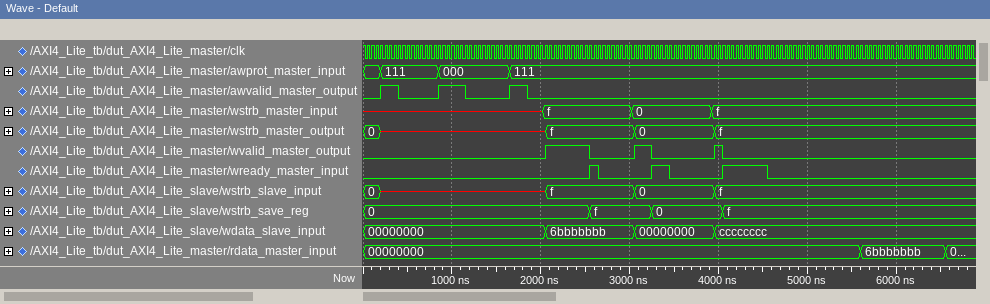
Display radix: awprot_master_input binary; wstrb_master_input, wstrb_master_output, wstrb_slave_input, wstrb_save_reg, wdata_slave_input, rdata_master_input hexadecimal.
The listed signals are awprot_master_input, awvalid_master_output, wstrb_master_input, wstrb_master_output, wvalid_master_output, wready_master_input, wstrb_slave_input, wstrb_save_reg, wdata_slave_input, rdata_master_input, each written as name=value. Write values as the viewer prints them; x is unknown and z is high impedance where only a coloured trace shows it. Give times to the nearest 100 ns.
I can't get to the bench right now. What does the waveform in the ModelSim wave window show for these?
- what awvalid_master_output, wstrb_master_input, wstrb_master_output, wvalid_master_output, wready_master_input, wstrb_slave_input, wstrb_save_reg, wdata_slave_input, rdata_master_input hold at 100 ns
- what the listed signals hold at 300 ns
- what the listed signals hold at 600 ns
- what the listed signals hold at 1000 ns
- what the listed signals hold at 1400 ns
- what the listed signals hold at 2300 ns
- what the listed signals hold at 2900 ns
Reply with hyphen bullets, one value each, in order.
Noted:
- awvalid_master_output=0, wstrb_master_input=x, wstrb_master_output=0, wvalid_master_output=0, wready_master_input=0, wstrb_slave_input=0, wstrb_save_reg=0, wdata_slave_input=00000000, rdata_master_input=00000000
- awprot_master_input=111, awvalid_master_output=1, wstrb_master_input=x, wstrb_master_output=x, wvalid_master_output=0, wready_master_input=0, wstrb_slave_input=x, wstrb_save_reg=0, wdata_slave_input=00000000, rdata_master_input=00000000
- awprot_master_input=111, awvalid_master_output=0, wstrb_master_input=x, wstrb_master_output=x, wvalid_master_output=0, wready_master_input=0, wstrb_slave_input=x, wstrb_save_reg=0, wdata_slave_input=00000000, rdata_master_input=00000000
- awprot_master_input=000, awvalid_master_output=1, wstrb_master_input=x, wstrb_master_output=x, wvalid_master_output=0, wready_master_input=0, wstrb_slave_input=x, wstrb_save_reg=0, wdata_slave_input=00000000, rdata_master_input=00000000
- awprot_master_input=000, awvalid_master_output=0, wstrb_master_input=x, wstrb_master_output=x, wvalid_master_output=0, wready_master_input=0, wstrb_slave_input=x, wstrb_save_reg=0, wdata_slave_input=00000000, rdata_master_input=00000000
- awprot_master_input=111, awvalid_master_output=0, wstrb_master_input=f, wstrb_master_output=f, wvalid_master_output=1, wready_master_input=0, wstrb_slave_input=f, wstrb_save_reg=0, wdata_slave_input=6bbbbbbb, rdata_master_input=00000000
- awprot_master_input=111, awvalid_master_output=0, wstrb_master_input=f, wstrb_master_output=f, wvalid_master_output=0, wready_master_input=0, wstrb_slave_input=f, wstrb_save_reg=f, wdata_slave_input=6bbbbbbb, rdata_master_input=00000000
